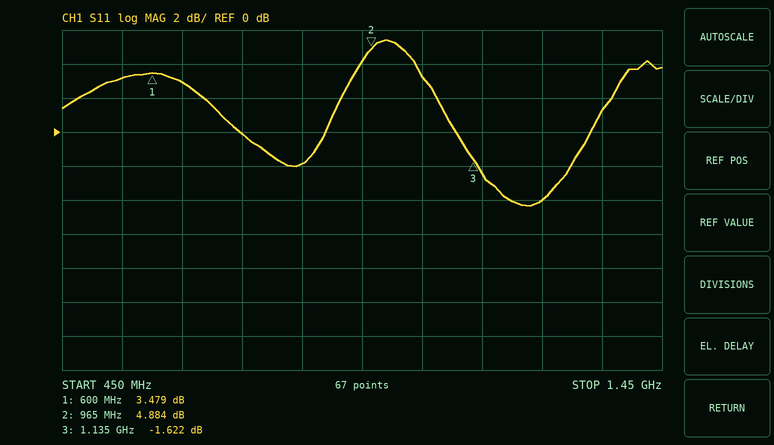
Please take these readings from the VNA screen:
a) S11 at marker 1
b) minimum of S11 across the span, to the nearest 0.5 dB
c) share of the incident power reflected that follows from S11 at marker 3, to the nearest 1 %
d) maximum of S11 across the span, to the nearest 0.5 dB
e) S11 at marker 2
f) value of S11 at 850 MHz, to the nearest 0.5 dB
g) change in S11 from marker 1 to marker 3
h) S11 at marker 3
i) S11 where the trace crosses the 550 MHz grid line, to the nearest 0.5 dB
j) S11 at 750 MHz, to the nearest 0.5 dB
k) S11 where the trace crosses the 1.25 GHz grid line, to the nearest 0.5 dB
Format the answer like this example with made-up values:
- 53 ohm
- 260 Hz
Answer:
- 3.479 dB
- -4.5 dB
- 69 %
- 5.5 dB
- 4.884 dB
- -2.0 dB
- -5.101 dB
- -1.622 dB
- 3.0 dB
- 0.0 dB
- -4.0 dB
